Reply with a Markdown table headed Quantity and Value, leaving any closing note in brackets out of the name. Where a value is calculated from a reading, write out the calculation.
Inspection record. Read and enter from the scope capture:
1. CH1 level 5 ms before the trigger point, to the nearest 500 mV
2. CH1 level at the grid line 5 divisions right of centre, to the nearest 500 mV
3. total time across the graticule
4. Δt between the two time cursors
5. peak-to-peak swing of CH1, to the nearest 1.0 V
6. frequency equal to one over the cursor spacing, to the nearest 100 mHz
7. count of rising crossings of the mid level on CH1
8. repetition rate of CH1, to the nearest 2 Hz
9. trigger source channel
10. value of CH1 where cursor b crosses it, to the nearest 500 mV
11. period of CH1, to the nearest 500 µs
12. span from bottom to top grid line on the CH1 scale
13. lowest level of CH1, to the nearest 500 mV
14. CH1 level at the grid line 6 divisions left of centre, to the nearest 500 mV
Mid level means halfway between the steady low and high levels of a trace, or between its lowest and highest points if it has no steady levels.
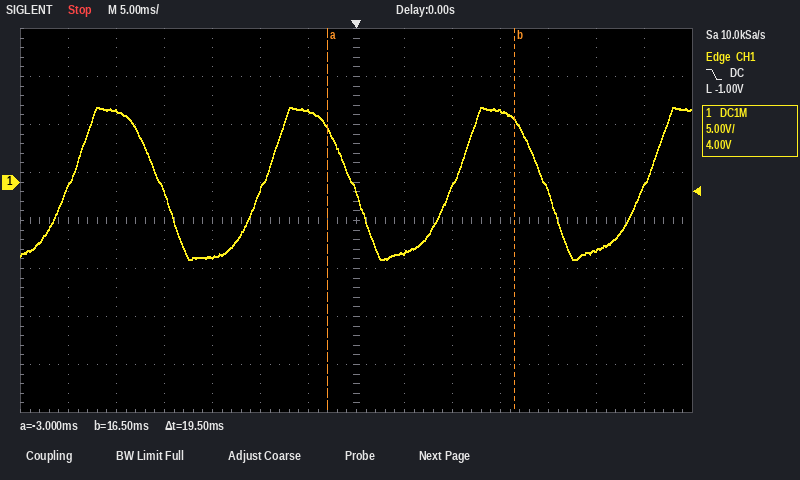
| Quantity | Value |
|---|---|
| CH1 level 5 ms before the trigger point, to the nearest 500 mV | 7.5 V |
| CH1 level at the grid line 5 divisions right of centre, to the nearest 500 mV | -7.0 V |
| total time across the graticule | 70 ms |
| Δt between the two time cursors | 19.5 ms |
| peak-to-peak swing of CH1, to the nearest 1.0 V | 16.0 V |
| frequency equal to one over the cursor spacing, to the nearest 100 mHz | 1 / 19.5 ms ≈ 51.3 Hz |
| count of rising crossings of the mid level on CH1 | 4 |
| repetition rate of CH1, to the nearest 2 Hz | 1 / 20.0 ms ≈ 50 Hz |
| trigger source channel | CH1 |
| value of CH1 where cursor b crosses it, to the nearest 500 mV | 6.5 V |
| period of CH1, to the nearest 500 µs | 20.0 ms |
| span from bottom to top grid line on the CH1 scale | 40 V |
| lowest level of CH1, to the nearest 500 mV | -8.0 V |
| CH1 level at the grid line 6 divisions left of centre, to the nearest 500 mV | -500 mV |
